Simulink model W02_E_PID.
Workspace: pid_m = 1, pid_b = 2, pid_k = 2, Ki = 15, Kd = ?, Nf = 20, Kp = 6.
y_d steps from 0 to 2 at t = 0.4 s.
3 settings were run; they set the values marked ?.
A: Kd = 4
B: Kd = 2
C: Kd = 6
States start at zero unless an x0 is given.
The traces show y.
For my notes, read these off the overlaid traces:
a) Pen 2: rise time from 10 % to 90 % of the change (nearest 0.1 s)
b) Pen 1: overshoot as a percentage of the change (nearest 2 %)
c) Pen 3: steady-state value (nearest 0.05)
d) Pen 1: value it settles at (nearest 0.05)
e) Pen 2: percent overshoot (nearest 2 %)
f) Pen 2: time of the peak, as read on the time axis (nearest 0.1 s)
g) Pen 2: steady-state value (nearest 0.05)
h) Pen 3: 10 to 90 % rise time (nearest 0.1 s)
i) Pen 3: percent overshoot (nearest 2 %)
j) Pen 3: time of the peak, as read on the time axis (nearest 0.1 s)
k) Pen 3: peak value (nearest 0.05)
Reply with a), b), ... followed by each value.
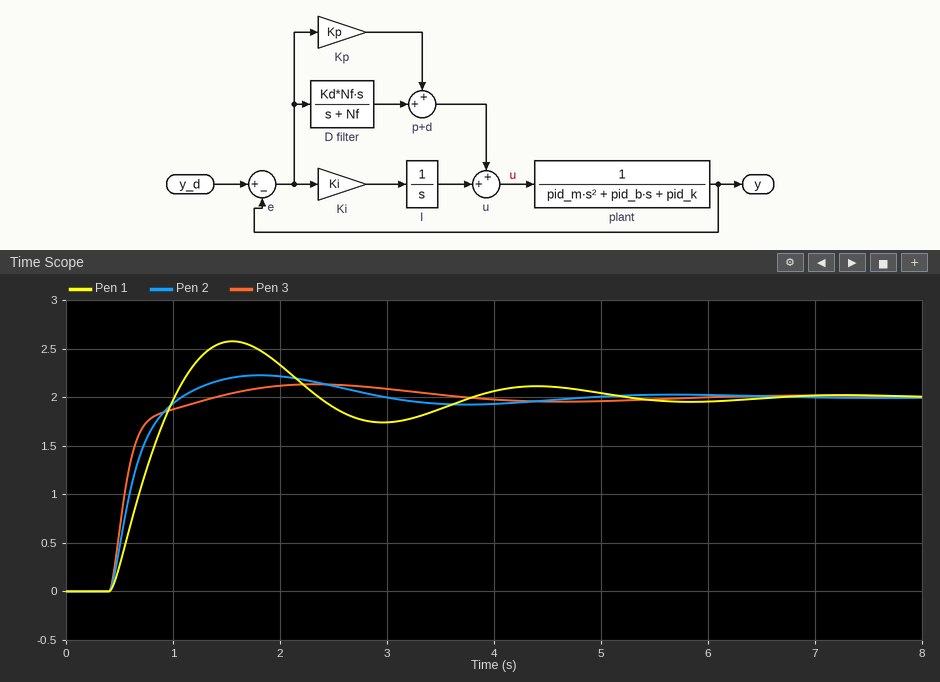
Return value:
a) 0.4 s
b) 28 %
c) 2.00
d) 2.00
e) 12 %
f) 1.8 s
g) 2.00
h) 0.4 s
i) 6 %
j) 2.3 s
k) 2.15
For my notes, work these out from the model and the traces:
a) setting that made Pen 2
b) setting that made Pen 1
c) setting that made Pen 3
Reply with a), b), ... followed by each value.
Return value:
a) A
b) B
c) C
